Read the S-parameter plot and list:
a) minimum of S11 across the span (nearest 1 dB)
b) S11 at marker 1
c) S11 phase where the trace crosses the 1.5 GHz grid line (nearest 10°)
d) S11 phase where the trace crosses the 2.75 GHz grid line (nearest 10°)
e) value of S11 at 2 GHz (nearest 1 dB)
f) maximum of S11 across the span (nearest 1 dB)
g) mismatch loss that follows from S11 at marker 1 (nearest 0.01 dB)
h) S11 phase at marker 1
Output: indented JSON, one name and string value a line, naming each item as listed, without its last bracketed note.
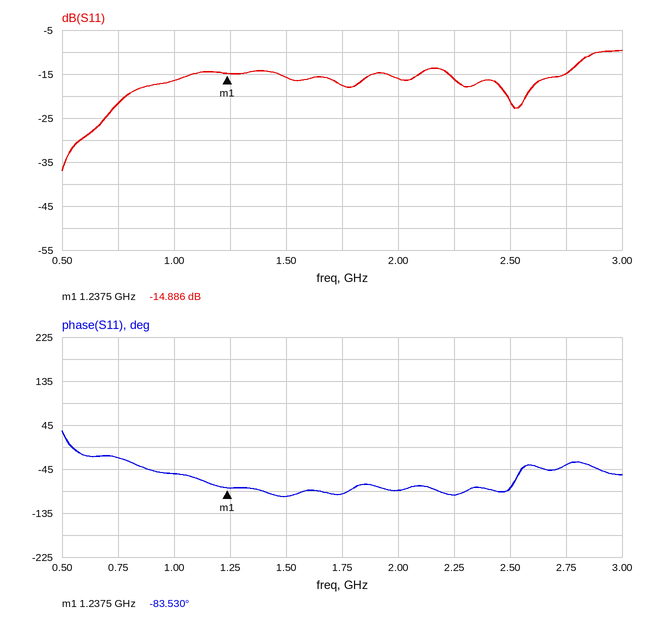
{
  "minimum of S11 across the span": "-37 dB",
  "S11 at marker 1": "-14.886 dB",
  "S11 phase where the trace crosses the 1.5 GHz grid line": "-100°",
  "S11 phase where the trace crosses the 2.75 GHz grid line": "-40°",
  "value of S11 at 2 GHz": "-16 dB",
  "maximum of S11 across the span": "-10 dB",
  "mismatch loss that follows from S11 at marker 1": "0.14 dB",
  "S11 phase at marker 1": "-83.530°"
}
